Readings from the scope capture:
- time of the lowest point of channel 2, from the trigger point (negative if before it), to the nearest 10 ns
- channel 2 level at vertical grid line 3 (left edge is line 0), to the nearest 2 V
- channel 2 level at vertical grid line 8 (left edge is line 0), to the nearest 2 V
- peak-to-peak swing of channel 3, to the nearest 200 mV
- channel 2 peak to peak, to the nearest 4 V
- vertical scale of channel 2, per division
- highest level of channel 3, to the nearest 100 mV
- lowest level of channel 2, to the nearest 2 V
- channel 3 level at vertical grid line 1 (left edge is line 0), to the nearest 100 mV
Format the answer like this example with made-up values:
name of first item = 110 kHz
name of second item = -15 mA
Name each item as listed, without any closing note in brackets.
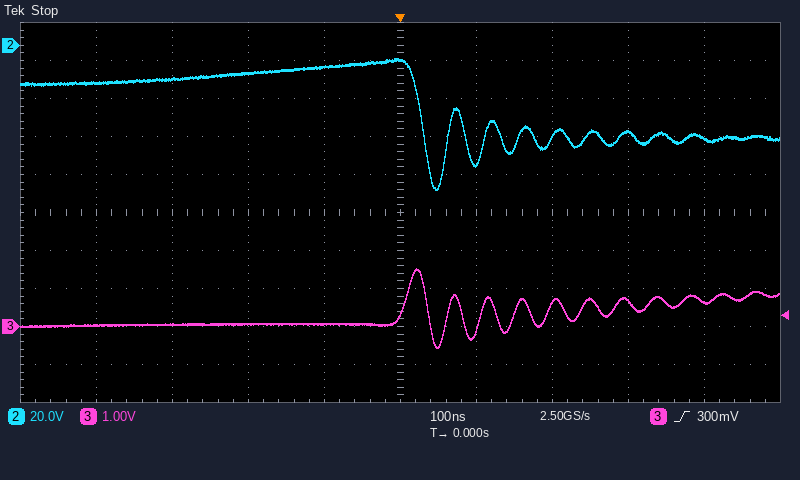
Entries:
time of the lowest point of channel 2, from the trigger point (negative if before it), to the nearest 10 ns = +50 ns
channel 2 level at vertical grid line 3 (left edge is line 0), to the nearest 2 V = -14 V
channel 2 level at vertical grid line 8 (left edge is line 0), to the nearest 2 V = -46 V
peak-to-peak swing of channel 3, to the nearest 200 mV = 2.0 V
channel 2 peak to peak, to the nearest 4 V = 68 V
vertical scale of channel 2, per division = 20 V
highest level of channel 3, to the nearest 100 mV = 1.5 V
lowest level of channel 2, to the nearest 2 V = -76 V
channel 3 level at vertical grid line 1 (left edge is line 0), to the nearest 100 mV = 0.0 V
